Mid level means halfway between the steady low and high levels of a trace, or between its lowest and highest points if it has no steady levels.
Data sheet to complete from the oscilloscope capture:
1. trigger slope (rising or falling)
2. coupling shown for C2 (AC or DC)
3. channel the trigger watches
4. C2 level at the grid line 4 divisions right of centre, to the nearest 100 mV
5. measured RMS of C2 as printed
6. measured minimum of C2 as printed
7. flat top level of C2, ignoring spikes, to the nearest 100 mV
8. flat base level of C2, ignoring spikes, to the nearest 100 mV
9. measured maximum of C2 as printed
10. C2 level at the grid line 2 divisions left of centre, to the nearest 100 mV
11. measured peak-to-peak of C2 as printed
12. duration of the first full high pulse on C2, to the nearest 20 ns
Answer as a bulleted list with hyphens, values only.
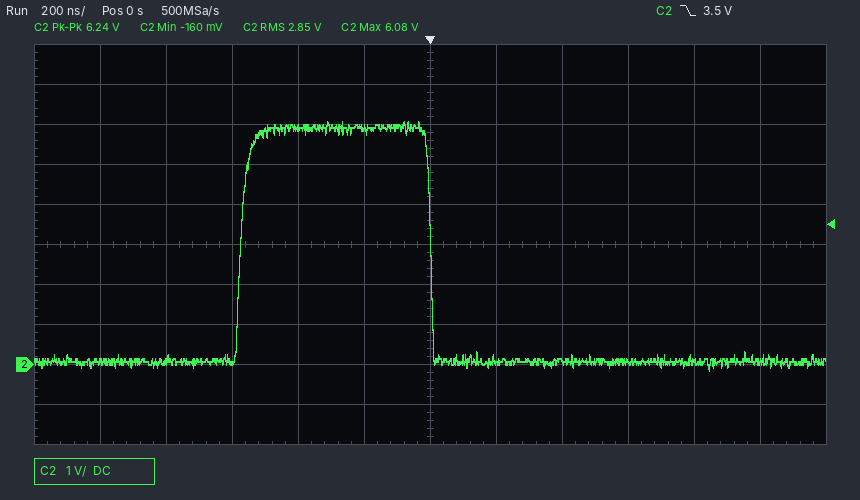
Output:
- falling
- DC
- C2
- 100 mV
- 2.85 V
- -160 mV
- 5.9 V
- 100 mV
- 6.08 V
- 5.9 V
- 6.24 V
- 580 ns
